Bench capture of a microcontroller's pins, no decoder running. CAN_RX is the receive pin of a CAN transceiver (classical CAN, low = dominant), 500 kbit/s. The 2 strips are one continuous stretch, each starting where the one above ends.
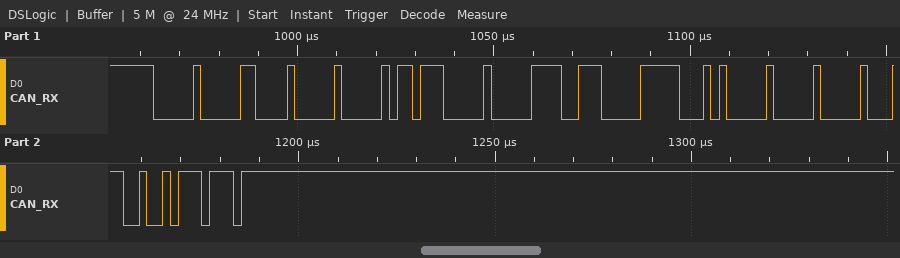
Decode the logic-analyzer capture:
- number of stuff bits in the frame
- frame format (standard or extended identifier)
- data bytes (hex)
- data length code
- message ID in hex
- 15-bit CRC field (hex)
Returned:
11
standard
00 DC 00 E7 07 94 00 00
8
0x002
0x64BB
